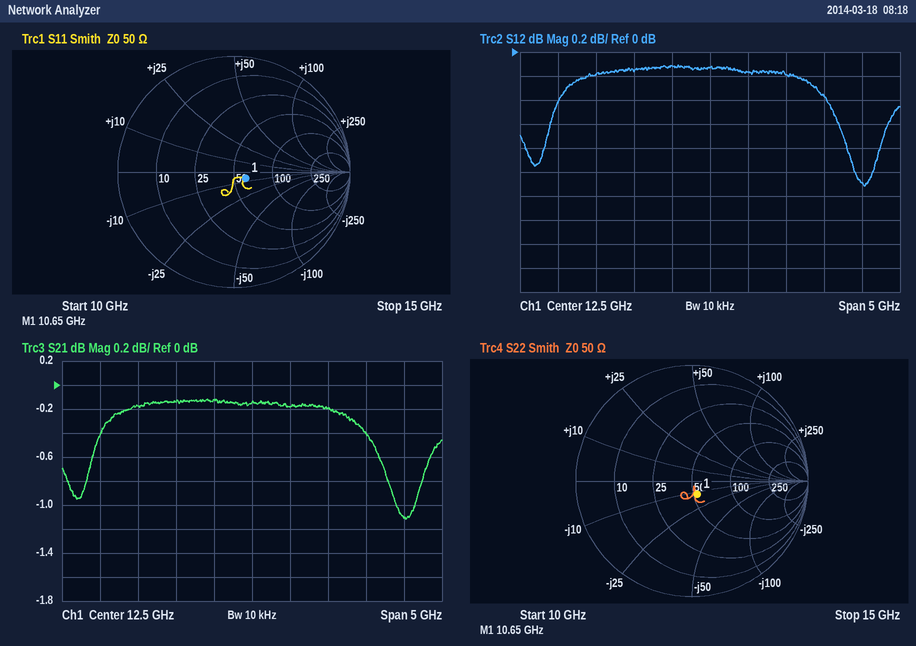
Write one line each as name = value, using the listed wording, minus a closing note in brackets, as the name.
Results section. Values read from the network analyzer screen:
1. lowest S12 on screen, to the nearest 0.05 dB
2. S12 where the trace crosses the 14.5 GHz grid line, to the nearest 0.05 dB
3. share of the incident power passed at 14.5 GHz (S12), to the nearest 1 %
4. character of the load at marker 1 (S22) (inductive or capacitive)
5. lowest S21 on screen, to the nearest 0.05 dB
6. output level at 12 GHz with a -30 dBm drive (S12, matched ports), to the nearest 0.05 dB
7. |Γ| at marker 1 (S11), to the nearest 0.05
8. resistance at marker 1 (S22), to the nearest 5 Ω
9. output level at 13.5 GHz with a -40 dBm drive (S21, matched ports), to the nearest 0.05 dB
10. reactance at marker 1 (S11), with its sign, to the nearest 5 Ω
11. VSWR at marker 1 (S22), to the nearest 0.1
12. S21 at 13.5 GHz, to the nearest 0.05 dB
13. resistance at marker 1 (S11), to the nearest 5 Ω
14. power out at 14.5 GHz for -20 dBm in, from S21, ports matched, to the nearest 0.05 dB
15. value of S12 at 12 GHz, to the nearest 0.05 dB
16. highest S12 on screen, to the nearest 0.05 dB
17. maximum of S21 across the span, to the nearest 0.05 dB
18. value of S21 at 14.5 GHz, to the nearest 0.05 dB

lowest S12 on screen, to the nearest 0.05 dB = -1.10 dB
S12 where the trace crosses the 14.5 GHz grid line, to the nearest 0.05 dB = -1.10 dB
share of the incident power passed at 14.5 GHz (S12), to the nearest 1 % = 78 %
character of the load at marker 1 (S22) = capacitive
lowest S21 on screen, to the nearest 0.05 dB = -1.10 dB
output level at 12 GHz with a -30 dBm drive (S12, matched ports), to the nearest 0.05 dB = -30.10 dBm
|Γ| at marker 1 (S11), to the nearest 0.05 = 0.10
resistance at marker 1 (S22), to the nearest 5 Ω = 55 Ω
output level at 13.5 GHz with a -40 dBm drive (S21, matched ports), to the nearest 0.05 dB = -40.20 dBm
reactance at marker 1 (S11), with its sign, to the nearest 5 Ω = -5 Ω
VSWR at marker 1 (S22), to the nearest 0.1 = 1.3
S21 at 13.5 GHz, to the nearest 0.05 dB = -0.20 dB
resistance at marker 1 (S11), to the nearest 5 Ω = 60 Ω
power out at 14.5 GHz for -20 dBm in, from S21, ports matched, to the nearest 0.05 dB = -21.10 dBm
value of S12 at 12 GHz, to the nearest 0.05 dB = -0.10 dB
highest S12 on screen, to the nearest 0.05 dB = -0.10 dB
maximum of S21 across the span, to the nearest 0.05 dB = -0.10 dB
value of S21 at 14.5 GHz, to the nearest 0.05 dB = -1.10 dB
